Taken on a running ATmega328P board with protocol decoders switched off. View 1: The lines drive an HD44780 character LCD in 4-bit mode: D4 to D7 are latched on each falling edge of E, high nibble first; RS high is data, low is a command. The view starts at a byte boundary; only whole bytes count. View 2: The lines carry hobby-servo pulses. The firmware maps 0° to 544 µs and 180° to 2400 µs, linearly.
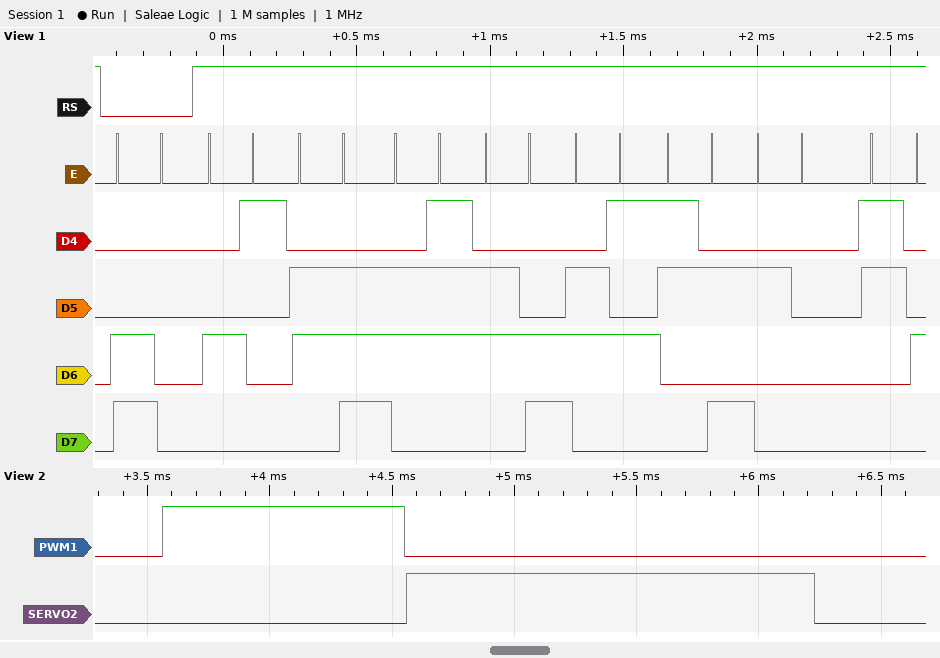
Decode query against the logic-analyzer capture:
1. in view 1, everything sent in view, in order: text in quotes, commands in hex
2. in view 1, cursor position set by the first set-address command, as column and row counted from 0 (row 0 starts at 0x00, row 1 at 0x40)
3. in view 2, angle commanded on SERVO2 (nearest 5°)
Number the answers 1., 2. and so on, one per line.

1. 0xC0 "Angle: 4"
2. column 0, row 1
3. 110°
